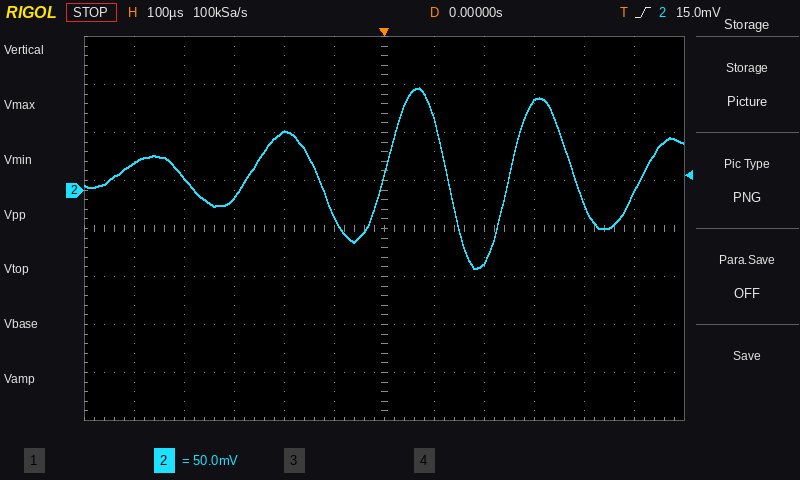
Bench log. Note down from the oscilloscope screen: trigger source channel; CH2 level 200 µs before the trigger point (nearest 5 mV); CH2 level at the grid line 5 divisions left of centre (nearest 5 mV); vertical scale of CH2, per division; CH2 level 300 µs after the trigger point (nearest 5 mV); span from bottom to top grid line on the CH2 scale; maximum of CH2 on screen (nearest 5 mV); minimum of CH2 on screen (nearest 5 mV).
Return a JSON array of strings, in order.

["CH2", "60 mV", "30 mV", "50 mV", "90 mV", "400 mV", "105 mV", "-80 mV"]
